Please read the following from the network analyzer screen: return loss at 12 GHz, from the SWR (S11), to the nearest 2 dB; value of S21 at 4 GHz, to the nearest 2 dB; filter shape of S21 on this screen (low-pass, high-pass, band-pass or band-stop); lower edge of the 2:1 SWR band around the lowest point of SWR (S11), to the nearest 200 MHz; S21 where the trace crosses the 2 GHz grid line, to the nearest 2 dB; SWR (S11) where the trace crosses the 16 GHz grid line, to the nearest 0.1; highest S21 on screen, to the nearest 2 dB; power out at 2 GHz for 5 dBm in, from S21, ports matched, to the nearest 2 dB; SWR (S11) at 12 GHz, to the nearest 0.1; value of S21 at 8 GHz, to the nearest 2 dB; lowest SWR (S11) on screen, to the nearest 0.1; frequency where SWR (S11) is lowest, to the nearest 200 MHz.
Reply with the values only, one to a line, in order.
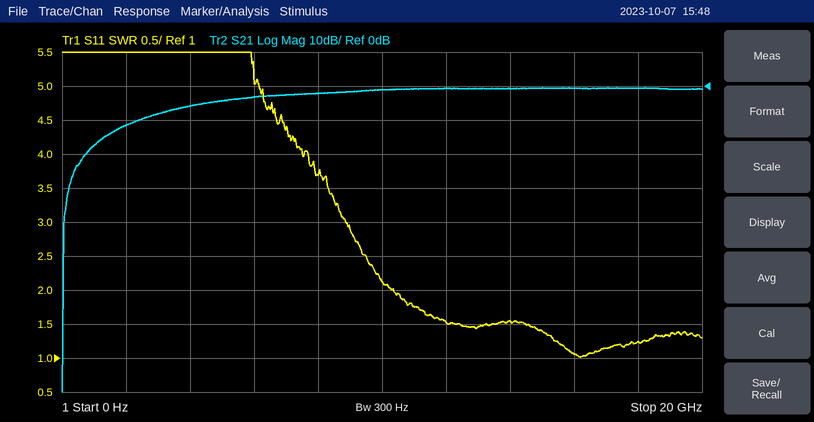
14 dB
-6 dB
high-pass
10.4 GHz
-12 dB
1.1
0 dB
-6 dBm
1.5
-2 dB
1.0
16.2 GHz
